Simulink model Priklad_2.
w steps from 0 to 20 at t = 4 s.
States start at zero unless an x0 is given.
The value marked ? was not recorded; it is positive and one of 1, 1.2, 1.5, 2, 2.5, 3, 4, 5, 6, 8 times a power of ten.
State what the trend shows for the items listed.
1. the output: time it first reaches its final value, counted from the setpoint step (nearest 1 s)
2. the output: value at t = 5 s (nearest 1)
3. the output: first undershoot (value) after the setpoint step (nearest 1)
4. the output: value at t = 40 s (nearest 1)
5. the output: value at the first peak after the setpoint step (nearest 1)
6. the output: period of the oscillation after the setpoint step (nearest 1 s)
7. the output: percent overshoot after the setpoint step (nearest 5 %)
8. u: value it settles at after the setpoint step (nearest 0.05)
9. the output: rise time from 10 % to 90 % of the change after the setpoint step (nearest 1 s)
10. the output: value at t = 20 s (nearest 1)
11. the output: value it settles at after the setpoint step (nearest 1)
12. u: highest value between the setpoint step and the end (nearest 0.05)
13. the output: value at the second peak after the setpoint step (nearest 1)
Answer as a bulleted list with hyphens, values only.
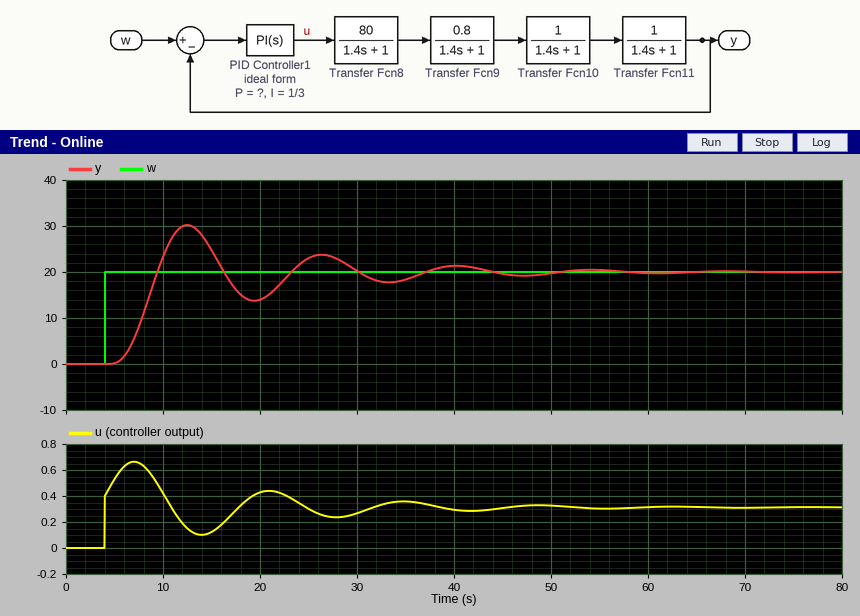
- 5 s
- 0
- 14
- 21
- 30
- 14 s
- 50 %
- 0.30
- 3 s
- 14
- 20
- 0.65
- 24
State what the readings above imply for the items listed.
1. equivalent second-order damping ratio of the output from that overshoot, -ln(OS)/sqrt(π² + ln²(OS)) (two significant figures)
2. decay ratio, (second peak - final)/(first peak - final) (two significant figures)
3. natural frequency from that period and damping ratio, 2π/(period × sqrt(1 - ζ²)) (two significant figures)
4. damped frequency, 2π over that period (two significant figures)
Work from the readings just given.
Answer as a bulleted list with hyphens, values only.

- 0.22
- 0.40
- 0.46 rad/s
- 0.45 rad/s
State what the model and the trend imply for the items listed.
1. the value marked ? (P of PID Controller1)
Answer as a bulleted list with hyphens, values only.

- 0.02
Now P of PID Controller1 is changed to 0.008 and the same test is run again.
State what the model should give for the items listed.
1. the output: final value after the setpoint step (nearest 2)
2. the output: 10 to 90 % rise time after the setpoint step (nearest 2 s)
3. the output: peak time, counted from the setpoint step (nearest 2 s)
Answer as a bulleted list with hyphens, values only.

- 20
- 6 s
- 14 s
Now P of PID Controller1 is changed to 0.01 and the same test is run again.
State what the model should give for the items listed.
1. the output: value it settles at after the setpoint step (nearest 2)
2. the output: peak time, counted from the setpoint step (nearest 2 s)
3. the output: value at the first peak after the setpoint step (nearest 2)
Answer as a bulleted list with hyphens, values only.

- 20
- 12 s
- 22
